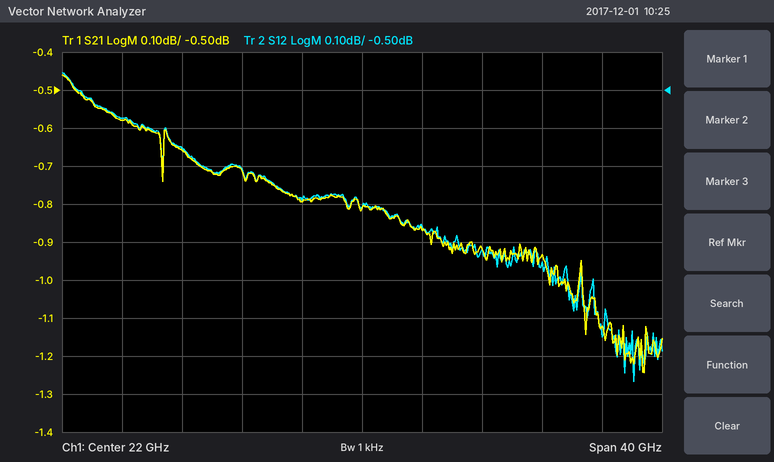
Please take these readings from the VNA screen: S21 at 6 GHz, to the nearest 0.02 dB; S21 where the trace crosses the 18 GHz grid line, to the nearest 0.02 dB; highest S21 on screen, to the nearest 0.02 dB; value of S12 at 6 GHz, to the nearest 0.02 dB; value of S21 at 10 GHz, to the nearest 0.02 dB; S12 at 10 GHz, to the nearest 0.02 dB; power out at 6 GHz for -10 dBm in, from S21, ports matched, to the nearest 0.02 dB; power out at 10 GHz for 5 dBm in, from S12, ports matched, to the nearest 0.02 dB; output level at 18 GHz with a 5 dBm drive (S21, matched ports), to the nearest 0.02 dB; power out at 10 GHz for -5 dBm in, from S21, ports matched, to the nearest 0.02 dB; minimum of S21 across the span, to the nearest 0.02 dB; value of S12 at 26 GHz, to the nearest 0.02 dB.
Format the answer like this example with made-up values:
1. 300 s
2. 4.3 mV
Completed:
1. -0.58 dB
2. -0.80 dB
3. -0.46 dB
4. -0.58 dB
5. -0.66 dB
6. -0.66 dB
7. -10.58 dBm
8. 4.34 dBm
9. 4.20 dBm
10. -5.66 dBm
11. -1.24 dB
12. -0.86 dB
